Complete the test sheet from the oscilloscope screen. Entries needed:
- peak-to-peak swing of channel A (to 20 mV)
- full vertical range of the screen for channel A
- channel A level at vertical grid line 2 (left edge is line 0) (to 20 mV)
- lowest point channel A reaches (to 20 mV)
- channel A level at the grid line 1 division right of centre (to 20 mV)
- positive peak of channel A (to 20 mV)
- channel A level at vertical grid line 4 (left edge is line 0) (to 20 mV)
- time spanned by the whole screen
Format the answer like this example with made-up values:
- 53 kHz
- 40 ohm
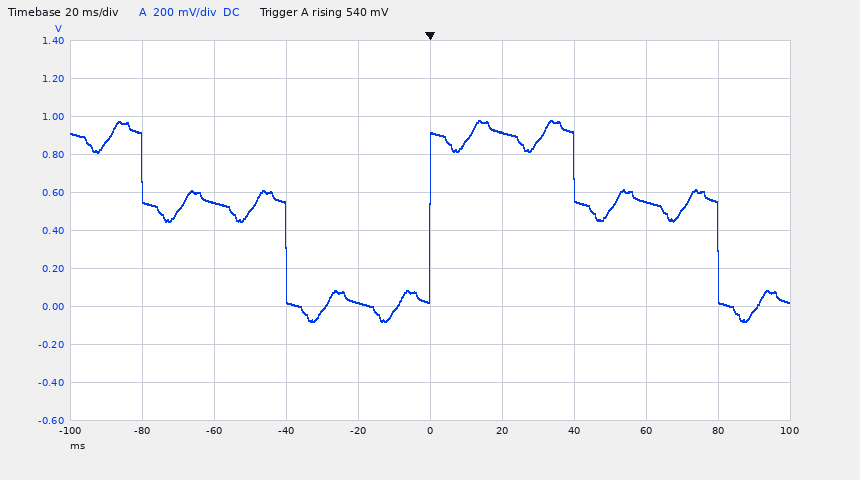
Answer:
- 1.06 V
- 2 V
- 540 mV
- -80 mV
- 920 mV
- 980 mV
- 20 mV
- 200 ms
